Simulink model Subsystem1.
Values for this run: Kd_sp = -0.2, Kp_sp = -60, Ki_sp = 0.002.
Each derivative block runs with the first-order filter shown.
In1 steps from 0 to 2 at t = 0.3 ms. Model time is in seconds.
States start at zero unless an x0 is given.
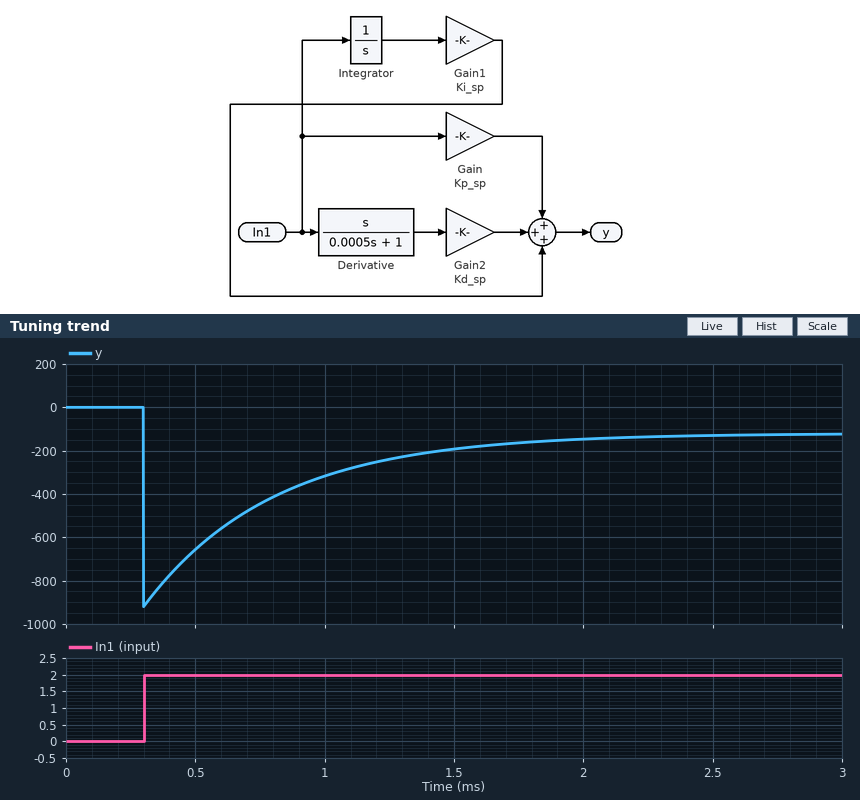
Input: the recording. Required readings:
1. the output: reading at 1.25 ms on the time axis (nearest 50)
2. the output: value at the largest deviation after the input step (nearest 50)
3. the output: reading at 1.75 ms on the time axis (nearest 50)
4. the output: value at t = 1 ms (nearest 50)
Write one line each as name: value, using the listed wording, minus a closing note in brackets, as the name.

the output: reading at 1.25 ms on the time axis: -250
the output: value at the largest deviation after the input step: -900
the output: reading at 1.75 ms on the time axis: -150
the output: value at t = 1 ms: -300
